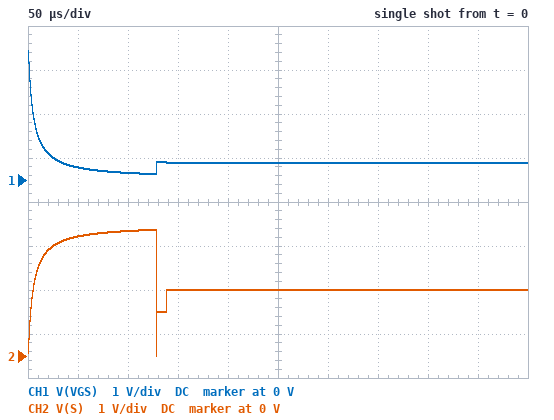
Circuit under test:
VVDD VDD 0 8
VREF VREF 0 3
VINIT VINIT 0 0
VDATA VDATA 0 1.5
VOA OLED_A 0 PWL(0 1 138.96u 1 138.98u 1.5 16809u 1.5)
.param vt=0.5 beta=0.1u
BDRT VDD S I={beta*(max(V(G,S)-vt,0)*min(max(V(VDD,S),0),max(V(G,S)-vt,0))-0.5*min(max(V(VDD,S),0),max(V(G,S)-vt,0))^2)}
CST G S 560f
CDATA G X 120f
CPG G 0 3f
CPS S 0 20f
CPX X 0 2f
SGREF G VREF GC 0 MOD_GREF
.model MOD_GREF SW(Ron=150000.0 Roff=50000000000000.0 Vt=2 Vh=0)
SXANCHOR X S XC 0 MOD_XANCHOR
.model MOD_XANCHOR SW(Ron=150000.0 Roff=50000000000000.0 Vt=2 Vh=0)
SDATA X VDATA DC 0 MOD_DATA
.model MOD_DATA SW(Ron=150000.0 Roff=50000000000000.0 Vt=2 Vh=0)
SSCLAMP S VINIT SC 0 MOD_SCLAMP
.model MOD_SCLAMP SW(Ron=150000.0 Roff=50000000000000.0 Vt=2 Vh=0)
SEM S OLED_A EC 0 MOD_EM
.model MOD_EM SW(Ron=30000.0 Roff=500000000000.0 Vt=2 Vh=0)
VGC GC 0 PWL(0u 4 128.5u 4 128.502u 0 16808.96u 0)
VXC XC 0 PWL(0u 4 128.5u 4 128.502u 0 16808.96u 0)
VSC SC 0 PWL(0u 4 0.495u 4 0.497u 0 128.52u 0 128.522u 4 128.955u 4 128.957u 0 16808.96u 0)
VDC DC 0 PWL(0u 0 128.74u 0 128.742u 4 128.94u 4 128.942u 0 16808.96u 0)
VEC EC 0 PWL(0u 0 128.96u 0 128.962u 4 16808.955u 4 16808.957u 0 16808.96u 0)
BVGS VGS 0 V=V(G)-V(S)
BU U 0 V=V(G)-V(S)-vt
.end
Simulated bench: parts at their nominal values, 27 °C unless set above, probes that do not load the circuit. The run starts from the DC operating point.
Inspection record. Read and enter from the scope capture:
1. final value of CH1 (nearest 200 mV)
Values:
400 mV
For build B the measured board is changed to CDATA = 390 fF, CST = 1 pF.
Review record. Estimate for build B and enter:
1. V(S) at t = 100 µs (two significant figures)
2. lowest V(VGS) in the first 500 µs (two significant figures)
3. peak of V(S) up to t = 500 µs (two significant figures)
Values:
2.7 V
230 mV
2.8 V
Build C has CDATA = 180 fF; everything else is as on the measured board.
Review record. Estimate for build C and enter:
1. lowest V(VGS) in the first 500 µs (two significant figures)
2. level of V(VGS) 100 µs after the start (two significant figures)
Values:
140 mV
170 mV
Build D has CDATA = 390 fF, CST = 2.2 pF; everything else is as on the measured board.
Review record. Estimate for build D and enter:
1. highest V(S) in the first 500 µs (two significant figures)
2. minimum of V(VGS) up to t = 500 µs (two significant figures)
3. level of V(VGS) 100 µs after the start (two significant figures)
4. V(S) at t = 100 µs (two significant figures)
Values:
2.6 V
380 mV
470 mV
2.5 V
